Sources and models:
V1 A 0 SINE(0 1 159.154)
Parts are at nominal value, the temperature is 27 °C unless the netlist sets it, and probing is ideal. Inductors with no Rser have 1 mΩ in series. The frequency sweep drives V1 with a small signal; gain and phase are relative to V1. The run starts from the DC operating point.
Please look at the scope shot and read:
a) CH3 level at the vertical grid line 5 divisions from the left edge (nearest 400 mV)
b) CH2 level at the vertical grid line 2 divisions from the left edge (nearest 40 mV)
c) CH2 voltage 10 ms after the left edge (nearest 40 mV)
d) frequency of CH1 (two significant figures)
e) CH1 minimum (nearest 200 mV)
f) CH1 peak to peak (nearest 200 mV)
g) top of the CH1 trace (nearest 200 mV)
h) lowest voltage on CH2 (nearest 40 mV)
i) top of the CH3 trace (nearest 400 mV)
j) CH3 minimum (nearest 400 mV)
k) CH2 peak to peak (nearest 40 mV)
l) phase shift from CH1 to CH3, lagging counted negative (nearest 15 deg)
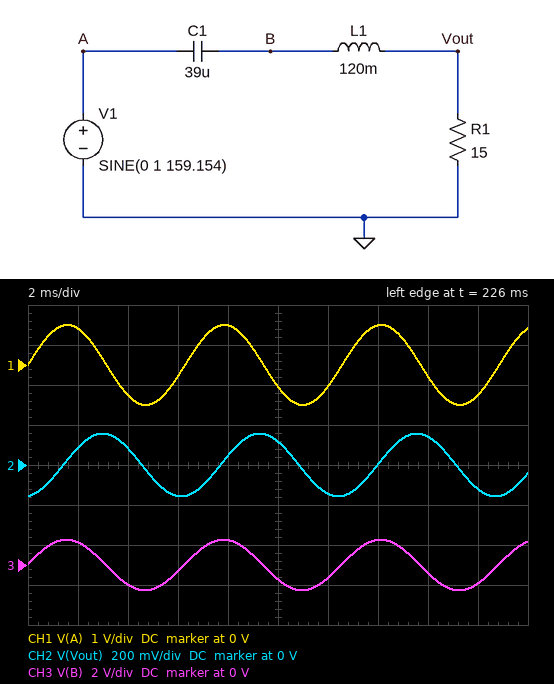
-800 mV
80 mV
120 mV
160 Hz
-1.0 V
2.0 V
1.0 V
-160 mV
1.2 V
-1.2 V
320 mV
0 deg
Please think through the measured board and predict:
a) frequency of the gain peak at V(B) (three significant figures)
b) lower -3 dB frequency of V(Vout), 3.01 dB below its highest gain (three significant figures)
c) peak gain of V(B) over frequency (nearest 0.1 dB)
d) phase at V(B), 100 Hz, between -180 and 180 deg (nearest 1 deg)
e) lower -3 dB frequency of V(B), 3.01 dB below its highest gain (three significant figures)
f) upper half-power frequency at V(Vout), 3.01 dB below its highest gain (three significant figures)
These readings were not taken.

74.9 Hz
64.3 Hz
11.7 dB
12 deg
66.2 Hz
84.2 Hz
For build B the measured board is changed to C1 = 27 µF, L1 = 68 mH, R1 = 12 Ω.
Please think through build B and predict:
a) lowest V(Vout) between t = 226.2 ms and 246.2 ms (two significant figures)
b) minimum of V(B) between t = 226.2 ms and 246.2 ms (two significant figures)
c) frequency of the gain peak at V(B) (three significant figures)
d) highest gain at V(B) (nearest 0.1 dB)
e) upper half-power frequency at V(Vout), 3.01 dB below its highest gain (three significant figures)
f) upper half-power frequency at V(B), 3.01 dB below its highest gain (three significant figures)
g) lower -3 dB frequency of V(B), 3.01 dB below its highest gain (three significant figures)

-360 mV
-2.1 V
119 Hz
12.7 dB
132 Hz
137 Hz
107 Hz
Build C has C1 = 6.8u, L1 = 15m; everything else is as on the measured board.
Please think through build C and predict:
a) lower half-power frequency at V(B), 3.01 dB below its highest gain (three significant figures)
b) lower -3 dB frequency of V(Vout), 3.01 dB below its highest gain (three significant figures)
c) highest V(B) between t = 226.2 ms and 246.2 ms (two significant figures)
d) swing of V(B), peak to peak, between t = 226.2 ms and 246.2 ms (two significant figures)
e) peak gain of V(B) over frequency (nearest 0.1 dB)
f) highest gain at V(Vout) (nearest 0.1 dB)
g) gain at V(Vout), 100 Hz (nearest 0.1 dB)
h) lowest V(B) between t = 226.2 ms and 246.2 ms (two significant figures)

442 Hz
425 Hz
160 mV
320 mV
10.4 dB
0 dB
-23.5 dB
-160 mV
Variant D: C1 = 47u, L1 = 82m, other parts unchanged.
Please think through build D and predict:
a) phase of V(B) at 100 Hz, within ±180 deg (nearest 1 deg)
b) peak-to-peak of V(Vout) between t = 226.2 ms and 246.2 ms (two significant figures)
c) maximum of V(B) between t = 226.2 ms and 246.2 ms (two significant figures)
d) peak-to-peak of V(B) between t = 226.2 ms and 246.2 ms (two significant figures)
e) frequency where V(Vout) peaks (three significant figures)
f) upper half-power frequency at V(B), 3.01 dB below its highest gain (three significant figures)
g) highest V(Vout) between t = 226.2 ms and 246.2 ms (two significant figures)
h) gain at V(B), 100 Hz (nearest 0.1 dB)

24 deg
480 mV
1.3 V
2.7 V
81.1 Hz
105 Hz
240 mV
7.3 dB
